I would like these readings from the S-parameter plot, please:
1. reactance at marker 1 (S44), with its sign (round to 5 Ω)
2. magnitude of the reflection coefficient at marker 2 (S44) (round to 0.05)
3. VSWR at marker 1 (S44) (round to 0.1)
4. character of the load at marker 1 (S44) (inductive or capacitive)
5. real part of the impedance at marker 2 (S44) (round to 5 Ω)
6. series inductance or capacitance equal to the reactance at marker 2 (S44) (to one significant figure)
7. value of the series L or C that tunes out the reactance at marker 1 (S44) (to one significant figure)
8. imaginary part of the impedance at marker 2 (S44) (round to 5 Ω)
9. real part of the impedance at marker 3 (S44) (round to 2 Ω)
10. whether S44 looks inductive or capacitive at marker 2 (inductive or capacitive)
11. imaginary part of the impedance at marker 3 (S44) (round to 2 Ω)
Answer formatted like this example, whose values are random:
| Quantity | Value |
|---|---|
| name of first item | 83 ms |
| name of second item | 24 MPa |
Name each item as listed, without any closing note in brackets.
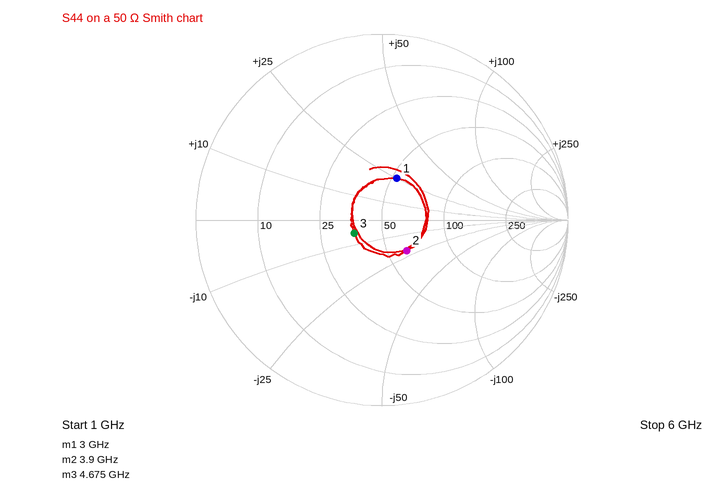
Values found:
| Quantity | Value |
|---|---|
| reactance at marker 1 (S44), with its sign | +25 Ω |
| magnitude of the reflection coefficient at marker 2 (S44) | 0.20 |
| VSWR at marker 1 (S44) | 1.6 |
| character of the load at marker 1 (S44) | inductive |
| real part of the impedance at marker 2 (S44) | 60 Ω |
| series inductance or capacitance equal to the reactance at marker 2 (S44) | 2 pF |
| value of the series L or C that tunes out the reactance at marker 1 (S44) | 2 pF |
| imaginary part of the impedance at marker 2 (S44) | -20 Ω |
| real part of the impedance at marker 3 (S44) | 36 Ω |
| whether S44 looks inductive or capacitive at marker 2 | capacitive |
| imaginary part of the impedance at marker 3 (S44) | -6 Ω |
